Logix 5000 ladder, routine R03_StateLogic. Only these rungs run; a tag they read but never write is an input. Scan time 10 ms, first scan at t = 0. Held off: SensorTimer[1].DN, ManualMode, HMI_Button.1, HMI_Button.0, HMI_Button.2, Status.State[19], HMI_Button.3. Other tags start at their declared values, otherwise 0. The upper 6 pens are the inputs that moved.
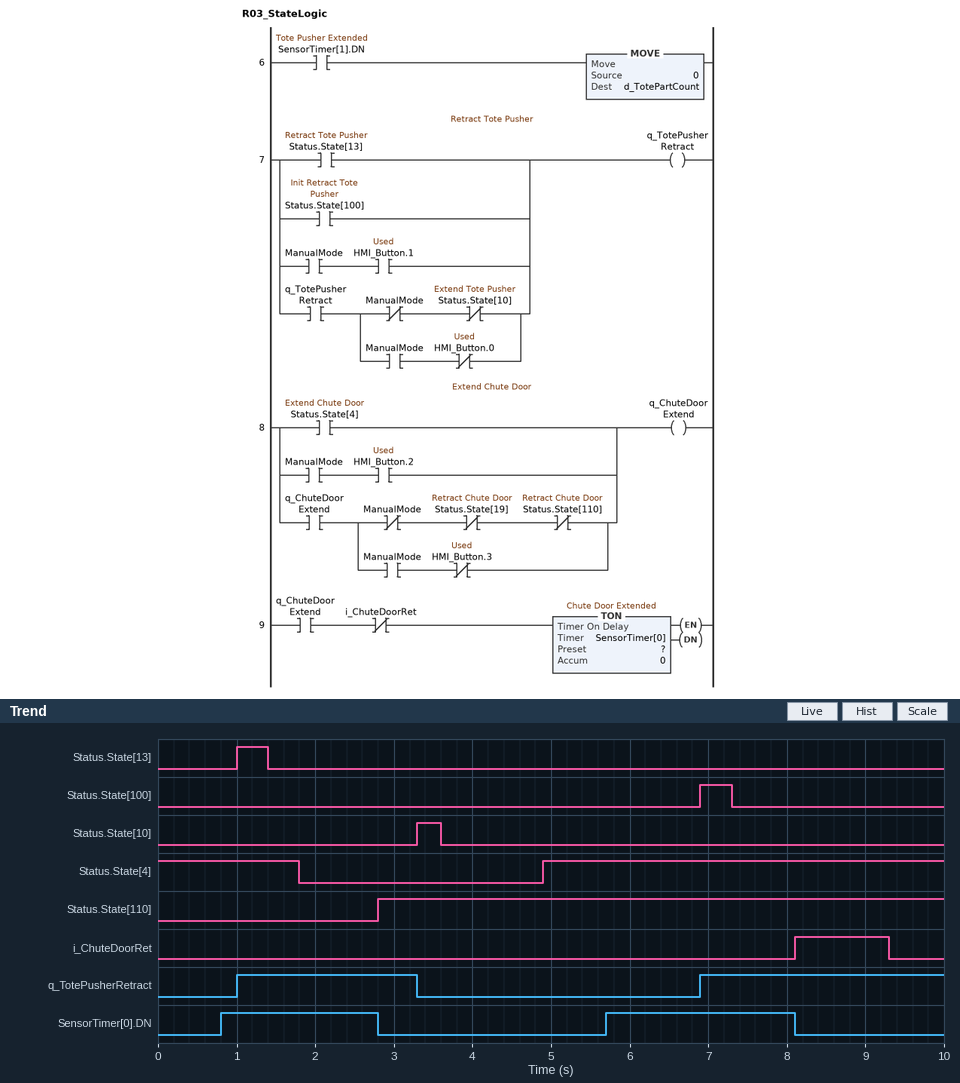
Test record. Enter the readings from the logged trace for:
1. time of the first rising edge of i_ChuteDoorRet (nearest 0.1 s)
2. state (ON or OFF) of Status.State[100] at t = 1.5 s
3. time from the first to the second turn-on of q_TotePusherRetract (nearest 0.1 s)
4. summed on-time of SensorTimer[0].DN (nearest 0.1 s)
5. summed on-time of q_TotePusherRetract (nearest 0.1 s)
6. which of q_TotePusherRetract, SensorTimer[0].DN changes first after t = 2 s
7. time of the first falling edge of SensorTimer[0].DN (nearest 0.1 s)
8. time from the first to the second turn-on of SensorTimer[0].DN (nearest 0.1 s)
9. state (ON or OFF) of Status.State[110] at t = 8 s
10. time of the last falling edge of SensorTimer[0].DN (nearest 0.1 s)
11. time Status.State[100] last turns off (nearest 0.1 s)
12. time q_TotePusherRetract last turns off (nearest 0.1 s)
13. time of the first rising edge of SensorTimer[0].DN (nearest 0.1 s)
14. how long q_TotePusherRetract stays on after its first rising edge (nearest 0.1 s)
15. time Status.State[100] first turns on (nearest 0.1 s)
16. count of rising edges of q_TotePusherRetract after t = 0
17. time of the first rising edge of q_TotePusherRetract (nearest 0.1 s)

8.1 s
OFF
5.9 s
4.4 s
5.4 s
SensorTimer[0].DN
2.8 s
4.9 s
ON
8.1 s
7.3 s
3.3 s
0.8 s
2.3 s
6.9 s
2
1.0 s
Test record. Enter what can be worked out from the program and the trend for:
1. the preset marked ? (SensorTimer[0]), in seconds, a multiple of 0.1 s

0.8 s
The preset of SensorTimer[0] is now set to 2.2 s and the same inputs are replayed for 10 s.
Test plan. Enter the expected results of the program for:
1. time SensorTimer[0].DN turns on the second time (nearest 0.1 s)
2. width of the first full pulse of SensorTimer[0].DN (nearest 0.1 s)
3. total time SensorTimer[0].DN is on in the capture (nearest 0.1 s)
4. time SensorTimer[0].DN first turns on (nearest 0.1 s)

7.1 s
0.6 s
1.6 s
2.2 s
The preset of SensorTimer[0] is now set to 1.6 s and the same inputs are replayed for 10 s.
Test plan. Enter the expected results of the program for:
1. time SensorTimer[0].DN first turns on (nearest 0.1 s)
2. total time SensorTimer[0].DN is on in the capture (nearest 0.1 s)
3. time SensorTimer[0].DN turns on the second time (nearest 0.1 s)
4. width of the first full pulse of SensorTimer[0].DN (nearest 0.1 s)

1.6 s
2.8 s
6.5 s
1.2 s
